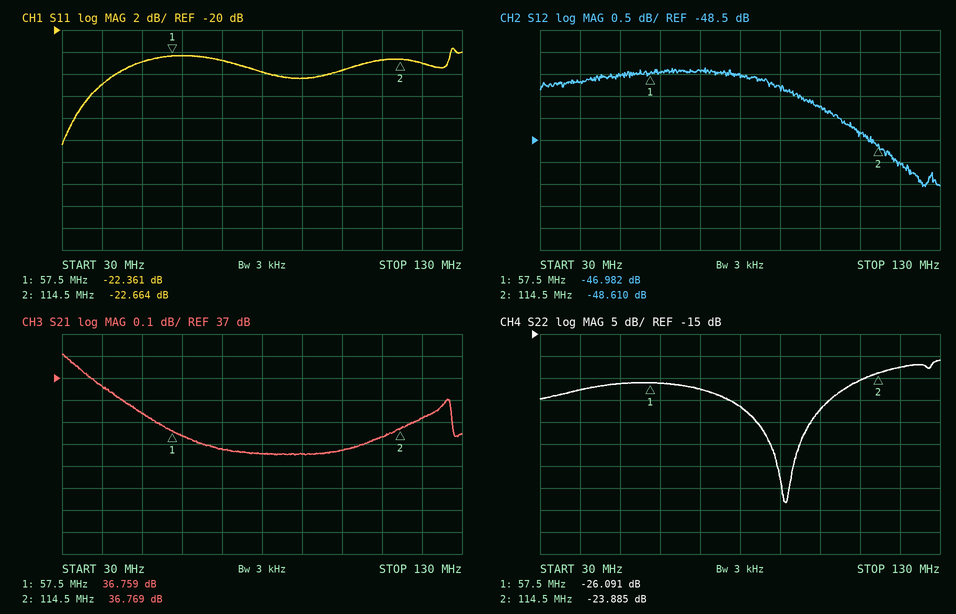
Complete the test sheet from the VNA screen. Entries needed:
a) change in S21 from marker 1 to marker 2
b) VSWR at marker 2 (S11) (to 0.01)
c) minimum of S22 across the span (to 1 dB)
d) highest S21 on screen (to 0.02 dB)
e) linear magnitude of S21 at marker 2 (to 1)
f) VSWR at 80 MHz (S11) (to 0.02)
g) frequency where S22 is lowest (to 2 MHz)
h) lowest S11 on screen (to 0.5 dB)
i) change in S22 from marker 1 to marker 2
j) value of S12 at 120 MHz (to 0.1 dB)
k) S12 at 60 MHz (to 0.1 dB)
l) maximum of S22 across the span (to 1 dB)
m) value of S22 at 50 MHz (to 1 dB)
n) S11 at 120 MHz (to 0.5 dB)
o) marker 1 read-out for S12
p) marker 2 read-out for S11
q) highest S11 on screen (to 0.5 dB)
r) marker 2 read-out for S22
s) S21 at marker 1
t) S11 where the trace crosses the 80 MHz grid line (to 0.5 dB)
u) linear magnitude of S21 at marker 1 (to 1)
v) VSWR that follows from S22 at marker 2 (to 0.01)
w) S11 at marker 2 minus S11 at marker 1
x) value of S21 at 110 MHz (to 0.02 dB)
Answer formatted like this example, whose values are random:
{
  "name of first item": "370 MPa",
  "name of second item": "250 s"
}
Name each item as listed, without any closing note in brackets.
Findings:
{
  "change in S21 from marker 1 to marker 2": "0.010 dB",
  "VSWR at marker 2 (S11)": "1.16",
  "minimum of S22 across the span": "-53 dB",
  "highest S21 on screen": "37.10 dB",
  "linear magnitude of S21 at marker 2": "69",
  "VSWR at 80 MHz (S11)": "1.14",
  "frequency where S22 is lowest": "92 MHz",
  "lowest S11 on screen": "-30.5 dB",
  "change in S22 from marker 1 to marker 2": "2.206 dB",
  "value of S12 at 120 MHz": "-49.0 dB",
  "S12 at 60 MHz": "-47.0 dB",
  "maximum of S22 across the span": "-21 dB",
  "value of S22 at 50 MHz": "-26 dB",
  "S11 at 120 MHz": "-23.0 dB",
  "marker 1 read-out for S12": "-46.982 dB",
  "marker 2 read-out for S11": "-22.664 dB",
  "highest S11 on screen": "-21.5 dB",
  "marker 2 read-out for S22": "-23.885 dB",
  "S21 at marker 1": "36.759 dB",
  "S11 where the trace crosses the 80 MHz grid line": "-24.0 dB",
  "linear magnitude of S21 at marker 1": "69",
  "VSWR that follows from S22 at marker 2": "1.14",
  "S11 at marker 2 minus S11 at marker 1": "-0.303 dB",
  "value of S21 at 110 MHz": "36.74 dB"
}
